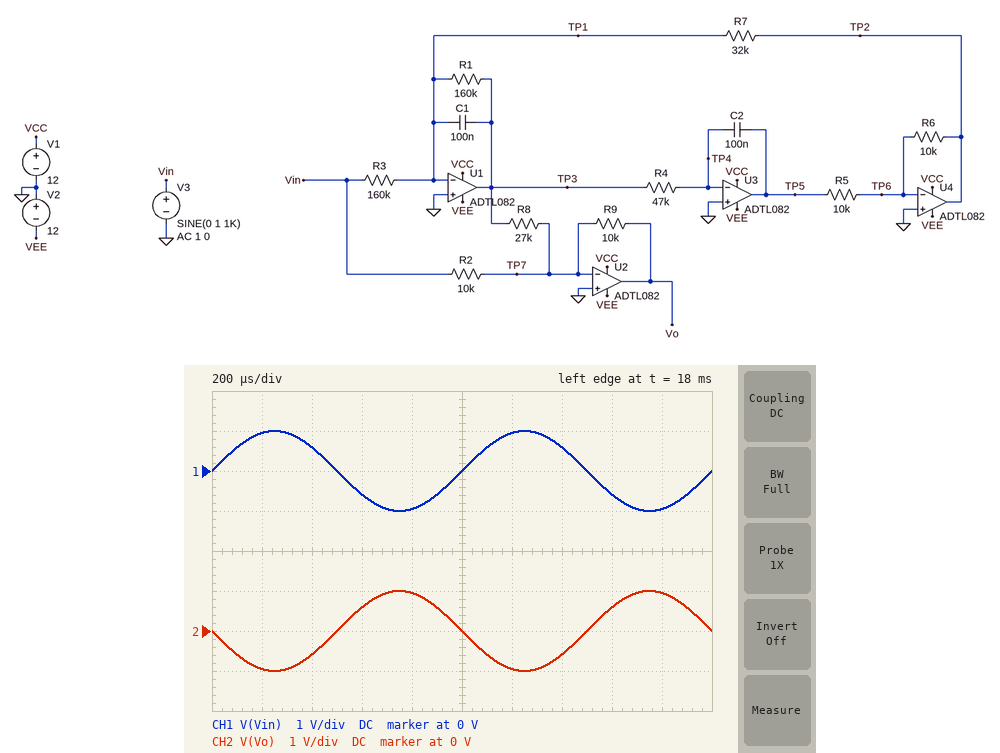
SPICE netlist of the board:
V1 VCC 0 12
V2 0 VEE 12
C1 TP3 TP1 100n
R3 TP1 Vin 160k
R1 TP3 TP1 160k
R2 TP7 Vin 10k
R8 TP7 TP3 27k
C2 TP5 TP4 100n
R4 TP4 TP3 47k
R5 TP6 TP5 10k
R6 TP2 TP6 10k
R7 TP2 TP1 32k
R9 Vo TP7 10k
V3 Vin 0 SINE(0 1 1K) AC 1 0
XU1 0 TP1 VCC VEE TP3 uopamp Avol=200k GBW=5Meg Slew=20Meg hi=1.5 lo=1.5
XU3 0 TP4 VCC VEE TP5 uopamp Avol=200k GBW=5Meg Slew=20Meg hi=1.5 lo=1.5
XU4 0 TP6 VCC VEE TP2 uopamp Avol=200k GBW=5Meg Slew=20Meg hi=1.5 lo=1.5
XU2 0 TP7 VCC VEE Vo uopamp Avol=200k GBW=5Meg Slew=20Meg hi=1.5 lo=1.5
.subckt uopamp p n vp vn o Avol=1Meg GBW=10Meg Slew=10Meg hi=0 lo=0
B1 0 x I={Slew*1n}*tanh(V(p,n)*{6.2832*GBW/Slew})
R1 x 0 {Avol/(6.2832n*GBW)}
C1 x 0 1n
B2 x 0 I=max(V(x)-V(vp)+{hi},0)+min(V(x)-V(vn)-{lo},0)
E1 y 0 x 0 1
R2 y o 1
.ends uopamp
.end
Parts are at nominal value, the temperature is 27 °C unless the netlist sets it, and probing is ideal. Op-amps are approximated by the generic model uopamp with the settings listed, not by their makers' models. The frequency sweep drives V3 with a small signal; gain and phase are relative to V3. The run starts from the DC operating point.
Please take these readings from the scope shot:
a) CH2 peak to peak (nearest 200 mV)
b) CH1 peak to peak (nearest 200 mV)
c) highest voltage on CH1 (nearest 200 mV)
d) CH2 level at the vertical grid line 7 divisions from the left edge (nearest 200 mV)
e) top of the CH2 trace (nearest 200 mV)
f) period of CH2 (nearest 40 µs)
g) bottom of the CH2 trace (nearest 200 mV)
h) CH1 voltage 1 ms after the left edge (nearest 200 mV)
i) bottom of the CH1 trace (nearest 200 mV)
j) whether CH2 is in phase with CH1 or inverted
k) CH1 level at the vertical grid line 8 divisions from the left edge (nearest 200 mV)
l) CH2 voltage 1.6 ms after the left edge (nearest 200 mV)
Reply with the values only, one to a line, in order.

2.0 V
2.0 V
1.0 V
-600 mV
1.0 V
1.00 ms
-1.0 V
0 V
-1.0 V
inverted
-600 mV
600 mV
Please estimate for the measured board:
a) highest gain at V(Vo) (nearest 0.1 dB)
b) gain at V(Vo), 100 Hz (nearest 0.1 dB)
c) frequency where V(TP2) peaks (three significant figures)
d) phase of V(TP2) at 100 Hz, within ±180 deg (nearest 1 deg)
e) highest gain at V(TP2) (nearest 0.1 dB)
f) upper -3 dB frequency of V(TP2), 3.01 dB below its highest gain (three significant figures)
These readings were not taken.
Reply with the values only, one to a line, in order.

0 dB
0 dB
40.4 Hz
7 deg
-1.6 dB
45.2 Hz
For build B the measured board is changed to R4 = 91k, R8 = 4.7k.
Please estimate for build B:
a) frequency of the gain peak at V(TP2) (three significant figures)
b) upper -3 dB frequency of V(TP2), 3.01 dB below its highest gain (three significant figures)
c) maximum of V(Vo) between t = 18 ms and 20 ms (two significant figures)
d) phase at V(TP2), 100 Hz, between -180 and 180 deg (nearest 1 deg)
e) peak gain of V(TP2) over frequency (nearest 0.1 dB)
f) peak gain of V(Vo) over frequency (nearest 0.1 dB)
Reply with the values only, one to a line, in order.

28.6 Hz
33.3 Hz
990 mV
6 deg
-4.4 dB
1.0 dB
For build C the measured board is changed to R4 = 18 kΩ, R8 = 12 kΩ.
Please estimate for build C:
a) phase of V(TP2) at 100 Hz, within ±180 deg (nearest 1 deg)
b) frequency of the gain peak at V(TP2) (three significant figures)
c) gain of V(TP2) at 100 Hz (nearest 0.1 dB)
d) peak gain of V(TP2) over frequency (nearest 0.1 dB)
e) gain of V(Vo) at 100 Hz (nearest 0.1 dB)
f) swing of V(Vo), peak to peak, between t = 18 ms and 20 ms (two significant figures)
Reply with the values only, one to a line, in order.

10 deg
65.9 Hz
-16.2 dB
2.5 dB
-0.1 dB
2.0 V
